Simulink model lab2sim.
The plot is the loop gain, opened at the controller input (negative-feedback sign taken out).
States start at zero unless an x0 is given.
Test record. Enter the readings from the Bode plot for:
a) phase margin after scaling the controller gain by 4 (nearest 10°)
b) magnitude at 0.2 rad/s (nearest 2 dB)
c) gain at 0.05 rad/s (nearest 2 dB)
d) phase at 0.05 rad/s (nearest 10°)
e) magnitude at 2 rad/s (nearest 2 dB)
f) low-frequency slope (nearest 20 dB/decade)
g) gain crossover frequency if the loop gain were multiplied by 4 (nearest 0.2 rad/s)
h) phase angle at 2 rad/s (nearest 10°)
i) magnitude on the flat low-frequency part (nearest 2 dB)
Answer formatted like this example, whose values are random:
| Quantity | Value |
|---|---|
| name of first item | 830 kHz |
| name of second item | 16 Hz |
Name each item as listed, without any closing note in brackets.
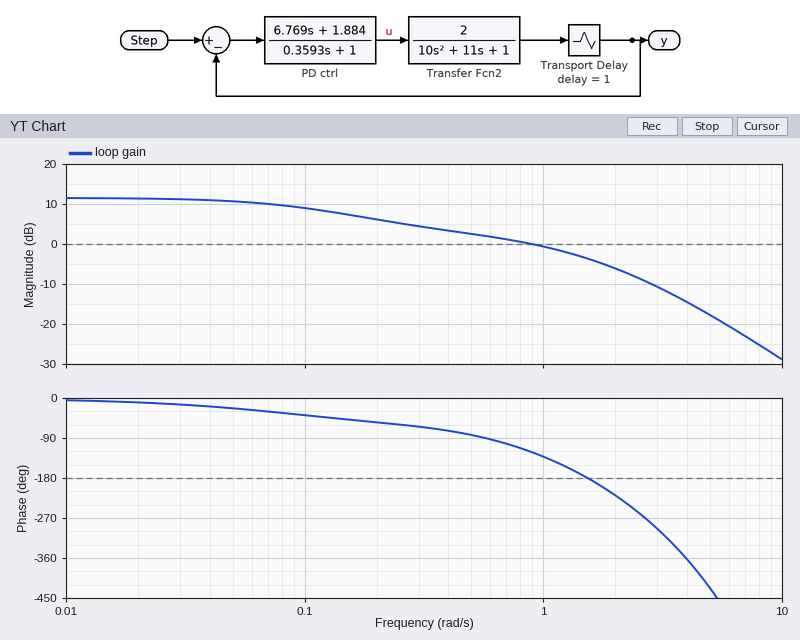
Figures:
| Quantity | Value |
|---|---|
| phase margin after scaling the controller gain by 4 | -140° |
| magnitude at 0.2 rad/s | 6 dB |
| gain at 0.05 rad/s | 10 dB |
| phase at 0.05 rad/s | -20° |
| magnitude at 2 rad/s | -6 dB |
| low-frequency slope | 0 dB/decade |
| gain crossover frequency if the loop gain were multiplied by 4 | 3.4 rad/s |
| phase angle at 2 rad/s | -220° |
| magnitude on the flat low-frequency part | 12 dB |
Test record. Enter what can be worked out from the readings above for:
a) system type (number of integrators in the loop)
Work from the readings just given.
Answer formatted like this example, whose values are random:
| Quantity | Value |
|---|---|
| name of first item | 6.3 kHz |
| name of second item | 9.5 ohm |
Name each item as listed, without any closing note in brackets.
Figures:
| Quantity | Value |
|---|---|
| system type | 0 |
